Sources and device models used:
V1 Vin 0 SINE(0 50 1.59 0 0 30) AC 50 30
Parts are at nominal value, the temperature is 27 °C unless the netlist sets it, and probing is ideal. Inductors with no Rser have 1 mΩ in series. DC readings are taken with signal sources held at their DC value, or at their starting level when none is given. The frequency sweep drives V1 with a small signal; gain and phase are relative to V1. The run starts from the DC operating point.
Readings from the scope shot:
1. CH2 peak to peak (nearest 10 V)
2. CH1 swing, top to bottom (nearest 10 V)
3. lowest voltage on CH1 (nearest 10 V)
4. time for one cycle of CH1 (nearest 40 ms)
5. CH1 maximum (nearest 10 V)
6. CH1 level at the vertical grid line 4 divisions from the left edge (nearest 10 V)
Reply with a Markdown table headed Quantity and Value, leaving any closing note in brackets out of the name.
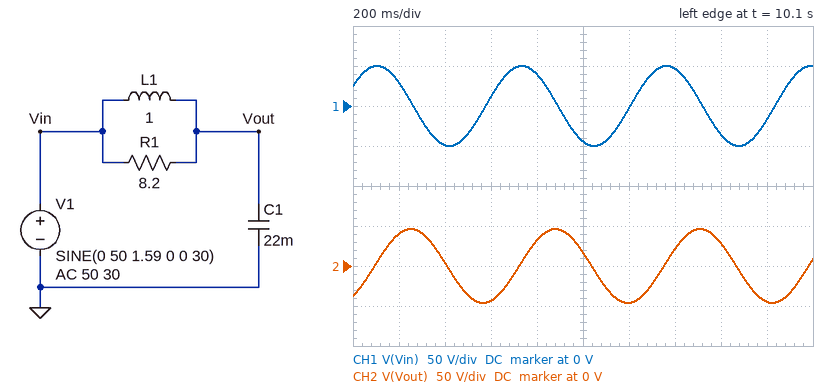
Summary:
| Quantity | Value |
|---|---|
| CH2 peak to peak | 90 V |
| CH1 swing, top to bottom | 100 V |
| lowest voltage on CH1 | -50 V |
| time for one cycle of CH1 | 640 ms |
| CH1 maximum | 50 V |
| CH1 level at the vertical grid line 4 divisions from the left edge | 40 V |
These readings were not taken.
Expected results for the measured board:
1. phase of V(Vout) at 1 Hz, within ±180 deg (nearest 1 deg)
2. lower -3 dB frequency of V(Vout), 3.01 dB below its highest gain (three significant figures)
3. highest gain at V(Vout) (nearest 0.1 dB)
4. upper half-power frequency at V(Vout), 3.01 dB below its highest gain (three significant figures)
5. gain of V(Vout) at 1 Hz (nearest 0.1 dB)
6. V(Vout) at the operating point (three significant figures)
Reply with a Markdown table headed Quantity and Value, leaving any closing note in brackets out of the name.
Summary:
| Quantity | Value |
|---|---|
| phase of V(Vout) at 1 Hz, within ±180 deg | -43 deg |
| lower -3 dB frequency of V(Vout), 3.01 dB below its highest gain | 410 mHz |
| highest gain at V(Vout) | 4.2 dB |
| upper half-power frequency at V(Vout), 3.01 dB below its highest gain | 1.39 Hz |
| gain of V(Vout) at 1 Hz | 4.2 dB |
| V(Vout) at the operating point | 25.0 V |
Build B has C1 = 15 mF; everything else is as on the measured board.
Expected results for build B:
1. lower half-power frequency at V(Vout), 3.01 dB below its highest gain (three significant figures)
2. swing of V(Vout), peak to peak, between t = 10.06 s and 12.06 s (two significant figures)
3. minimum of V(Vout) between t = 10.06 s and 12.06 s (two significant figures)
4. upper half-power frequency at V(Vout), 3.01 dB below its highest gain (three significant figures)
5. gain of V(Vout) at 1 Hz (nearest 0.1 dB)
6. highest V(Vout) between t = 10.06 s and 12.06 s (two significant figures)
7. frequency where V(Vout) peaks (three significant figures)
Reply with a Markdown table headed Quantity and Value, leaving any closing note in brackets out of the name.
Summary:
| Quantity | Value |
|---|---|
| lower half-power frequency at V(Vout), 3.01 dB below its highest gain | 260 mHz |
| swing of V(Vout), peak to peak, between t = 10.06 s and 12.06 s | 120 V |
| minimum of V(Vout) between t = 10.06 s and 12.06 s | -60 V |
| upper half-power frequency at V(Vout), 3.01 dB below its highest gain | 1.78 Hz |
| gain of V(Vout) at 1 Hz | 3.2 dB |
| highest V(Vout) between t = 10.06 s and 12.06 s | 60 V |
| frequency where V(Vout) peaks | 1.11 Hz |
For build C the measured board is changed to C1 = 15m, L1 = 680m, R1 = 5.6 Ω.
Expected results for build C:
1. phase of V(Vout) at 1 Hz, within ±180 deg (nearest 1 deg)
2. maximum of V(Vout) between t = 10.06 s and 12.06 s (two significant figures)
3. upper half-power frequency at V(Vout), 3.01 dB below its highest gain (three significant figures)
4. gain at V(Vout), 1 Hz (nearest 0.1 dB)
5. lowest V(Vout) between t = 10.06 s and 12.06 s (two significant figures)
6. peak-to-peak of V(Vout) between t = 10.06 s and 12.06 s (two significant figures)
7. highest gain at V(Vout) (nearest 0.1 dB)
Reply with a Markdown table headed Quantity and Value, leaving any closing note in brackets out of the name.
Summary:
| Quantity | Value |
|---|---|
| phase of V(Vout) at 1 Hz, within ±180 deg | -15 deg |
| maximum of V(Vout) between t = 10.06 s and 12.06 s | 65 V |
| upper half-power frequency at V(Vout), 3.01 dB below its highest gain | 2.33 Hz |
| gain at V(Vout), 1 Hz | 2.3 dB |
| lowest V(Vout) between t = 10.06 s and 12.06 s | -65 V |
| peak-to-peak of V(Vout) between t = 10.06 s and 12.06 s | 130 V |
| highest gain at V(Vout) | 2.6 dB |
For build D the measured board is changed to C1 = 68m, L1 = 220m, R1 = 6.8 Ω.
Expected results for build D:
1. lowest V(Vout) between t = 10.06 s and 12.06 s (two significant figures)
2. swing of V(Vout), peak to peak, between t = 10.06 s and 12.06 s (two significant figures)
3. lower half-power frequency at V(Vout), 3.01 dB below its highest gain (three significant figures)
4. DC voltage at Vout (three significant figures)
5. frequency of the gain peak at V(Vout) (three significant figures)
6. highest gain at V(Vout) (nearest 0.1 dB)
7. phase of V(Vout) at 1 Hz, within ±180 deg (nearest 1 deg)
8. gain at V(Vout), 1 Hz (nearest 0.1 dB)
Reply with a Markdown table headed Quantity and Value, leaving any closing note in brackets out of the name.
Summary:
| Quantity | Value |
|---|---|
| lowest V(Vout) between t = 10.06 s and 12.06 s | -89 V |
| swing of V(Vout), peak to peak, between t = 10.06 s and 12.06 s | 180 V |
| lower half-power frequency at V(Vout), 3.01 dB below its highest gain | 1.09 Hz |
| DC voltage at Vout | 25.0 V |
| frequency of the gain peak at V(Vout) | 1.28 Hz |
| highest gain at V(Vout) | 11.9 dB |
| phase of V(Vout) at 1 Hz, within ±180 deg | -15 deg |
| gain at V(Vout), 1 Hz | 7.0 dB |
